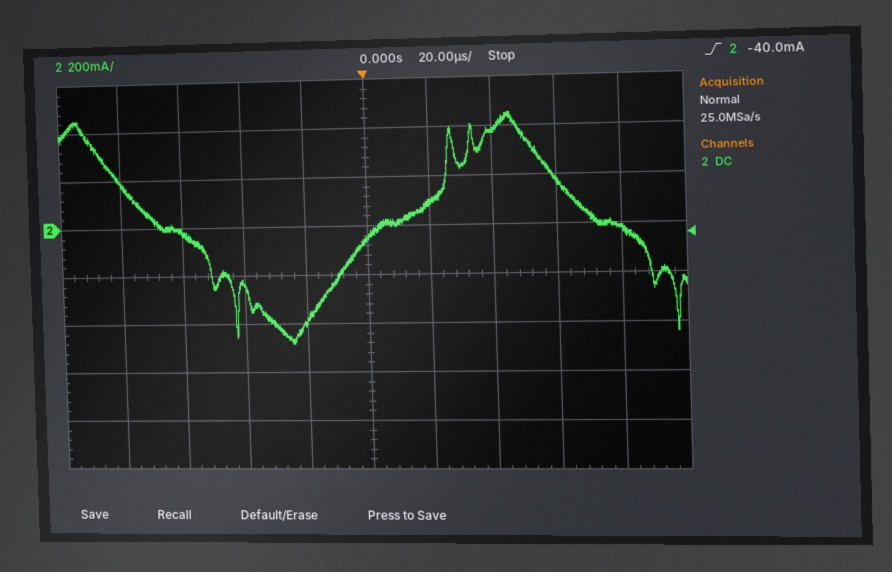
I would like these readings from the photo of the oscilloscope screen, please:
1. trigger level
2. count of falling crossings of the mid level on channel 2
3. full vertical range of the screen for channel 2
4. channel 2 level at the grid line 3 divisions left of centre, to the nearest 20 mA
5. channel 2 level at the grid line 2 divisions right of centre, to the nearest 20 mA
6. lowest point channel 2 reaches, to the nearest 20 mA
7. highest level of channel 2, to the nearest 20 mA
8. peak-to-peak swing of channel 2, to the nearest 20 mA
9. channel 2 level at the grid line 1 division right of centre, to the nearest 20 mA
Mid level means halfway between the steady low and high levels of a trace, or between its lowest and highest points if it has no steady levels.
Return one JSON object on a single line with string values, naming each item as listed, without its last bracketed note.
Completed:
{"trigger level": "-40.0 mA", "count of falling crossings of the mid level on channel 2": "2", "full vertical range of the screen for channel 2": "1.6 A", "channel 2 level at the grid line 3 divisions left of centre, to the nearest 20 mA": "-20 mA", "channel 2 level at the grid line 2 divisions right of centre, to the nearest 20 mA": "380 mA", "lowest point channel 2 reaches, to the nearest 20 mA": "-480 mA", "highest level of channel 2, to the nearest 20 mA": "460 mA", "peak-to-peak swing of channel 2, to the nearest 20 mA": "940 mA", "channel 2 level at the grid line 1 division right of centre, to the nearest 20 mA": "100 mA"}
